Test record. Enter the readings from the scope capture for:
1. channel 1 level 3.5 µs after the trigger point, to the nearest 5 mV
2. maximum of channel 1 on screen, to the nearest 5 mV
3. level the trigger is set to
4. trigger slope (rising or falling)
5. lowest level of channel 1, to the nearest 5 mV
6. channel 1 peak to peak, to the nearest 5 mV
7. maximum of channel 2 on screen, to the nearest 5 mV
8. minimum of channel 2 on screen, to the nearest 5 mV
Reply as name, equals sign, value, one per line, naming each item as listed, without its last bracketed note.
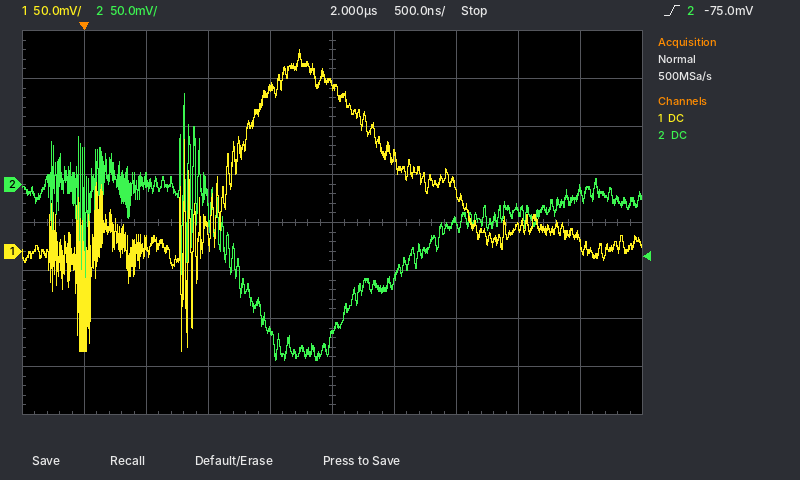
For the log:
channel 1 level 3.5 µs after the trigger point, to the nearest 5 mV = 25 mV
maximum of channel 1 on screen, to the nearest 5 mV = 210 mV
level the trigger is set to = -75.0 mV
trigger slope = rising
lowest level of channel 1, to the nearest 5 mV = -105 mV
channel 1 peak to peak, to the nearest 5 mV = 315 mV
maximum of channel 2 on screen, to the nearest 5 mV = 95 mV
minimum of channel 2 on screen, to the nearest 5 mV = -185 mV
